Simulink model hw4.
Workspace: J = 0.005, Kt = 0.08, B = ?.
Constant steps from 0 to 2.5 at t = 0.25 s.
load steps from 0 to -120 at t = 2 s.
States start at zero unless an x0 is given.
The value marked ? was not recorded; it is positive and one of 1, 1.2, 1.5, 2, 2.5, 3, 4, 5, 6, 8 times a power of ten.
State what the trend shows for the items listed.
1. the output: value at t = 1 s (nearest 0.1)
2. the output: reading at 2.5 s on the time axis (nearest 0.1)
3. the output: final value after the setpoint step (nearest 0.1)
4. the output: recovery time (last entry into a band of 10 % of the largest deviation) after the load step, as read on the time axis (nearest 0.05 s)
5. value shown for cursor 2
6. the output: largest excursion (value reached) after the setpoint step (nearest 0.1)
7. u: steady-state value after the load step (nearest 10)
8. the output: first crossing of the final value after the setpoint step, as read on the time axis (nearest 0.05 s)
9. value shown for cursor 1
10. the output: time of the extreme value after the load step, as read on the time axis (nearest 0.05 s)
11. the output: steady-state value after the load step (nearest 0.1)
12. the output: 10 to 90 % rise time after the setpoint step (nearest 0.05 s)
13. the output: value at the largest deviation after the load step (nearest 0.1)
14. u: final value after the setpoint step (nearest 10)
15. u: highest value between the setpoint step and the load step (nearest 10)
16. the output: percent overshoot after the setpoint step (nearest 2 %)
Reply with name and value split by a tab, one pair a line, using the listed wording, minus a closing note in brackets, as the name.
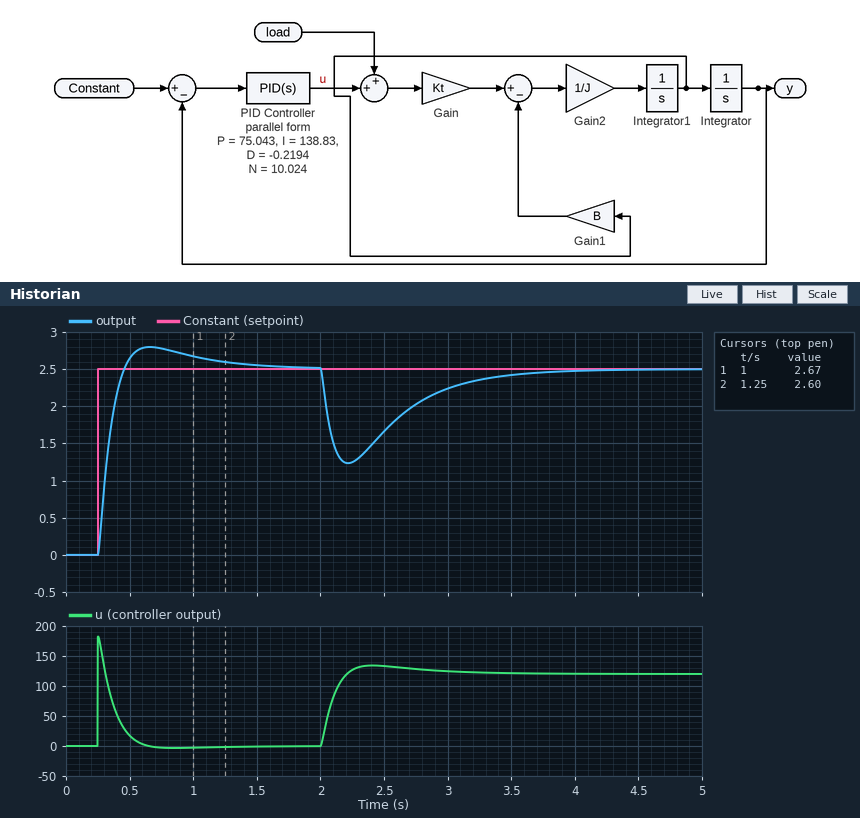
the output: value at t = 1 s	2.7
the output: reading at 2.5 s on the time axis	1.7
the output: final value after the setpoint step	2.5
the output: recovery time (last entry into a band of 10 % of the largest deviation) after the load step, as read on the time axis	3.30 s
value shown for cursor 2	2.60
the output: largest excursion (value reached) after the setpoint step	2.8
u: steady-state value after the load step	120
the output: first crossing of the final value after the setpoint step, as read on the time axis	0.45 s
value shown for cursor 1	2.67
the output: time of the extreme value after the load step, as read on the time axis	2.20 s
the output: steady-state value after the load step	2.5
the output: 10 to 90 % rise time after the setpoint step	0.15 s
the output: value at the largest deviation after the load step	1.2
u: final value after the setpoint step	0
u: highest value between the setpoint step and the load step	180
the output: percent overshoot after the setpoint step	12 %
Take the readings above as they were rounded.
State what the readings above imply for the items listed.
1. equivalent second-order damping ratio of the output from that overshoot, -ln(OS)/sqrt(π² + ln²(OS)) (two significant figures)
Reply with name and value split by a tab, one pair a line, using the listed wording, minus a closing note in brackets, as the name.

equivalent second-order damping ratio of the output from that overshoot, -ln(OS)/sqrt(π² + ln²(OS))	0.56
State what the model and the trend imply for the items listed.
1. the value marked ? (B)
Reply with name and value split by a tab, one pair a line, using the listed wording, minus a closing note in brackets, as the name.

the value marked ?	0.6
